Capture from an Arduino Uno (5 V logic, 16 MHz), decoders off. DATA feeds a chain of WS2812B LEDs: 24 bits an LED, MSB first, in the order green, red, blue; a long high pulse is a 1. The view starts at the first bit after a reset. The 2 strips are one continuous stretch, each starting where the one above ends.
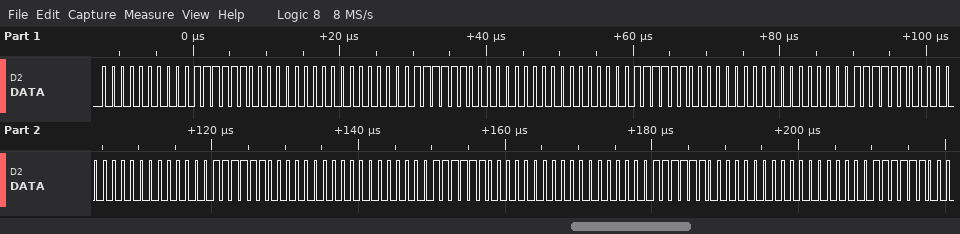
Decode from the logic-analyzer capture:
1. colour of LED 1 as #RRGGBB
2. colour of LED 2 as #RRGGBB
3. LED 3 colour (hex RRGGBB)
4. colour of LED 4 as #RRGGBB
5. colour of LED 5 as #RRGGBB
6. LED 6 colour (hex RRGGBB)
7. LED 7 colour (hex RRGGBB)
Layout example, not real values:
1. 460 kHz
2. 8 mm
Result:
1. #3F0000
2. #3F0000
3. #3F0000
4. #3F0000
5. #3F0000
6. #3F0000
7. #3F0000
